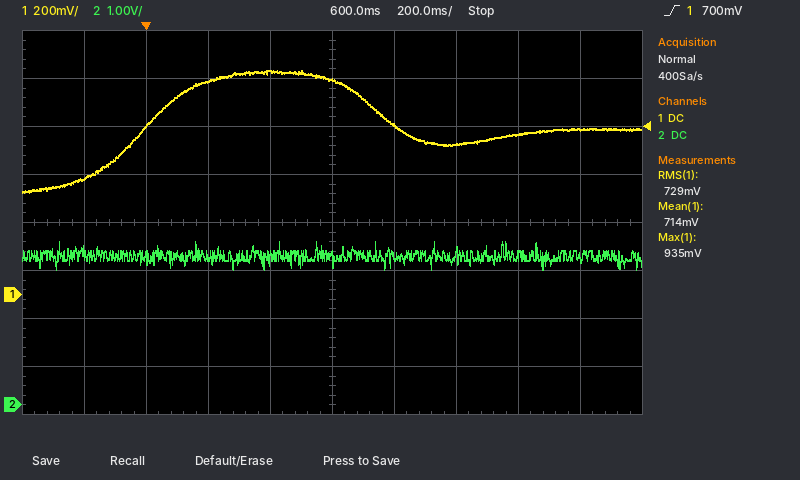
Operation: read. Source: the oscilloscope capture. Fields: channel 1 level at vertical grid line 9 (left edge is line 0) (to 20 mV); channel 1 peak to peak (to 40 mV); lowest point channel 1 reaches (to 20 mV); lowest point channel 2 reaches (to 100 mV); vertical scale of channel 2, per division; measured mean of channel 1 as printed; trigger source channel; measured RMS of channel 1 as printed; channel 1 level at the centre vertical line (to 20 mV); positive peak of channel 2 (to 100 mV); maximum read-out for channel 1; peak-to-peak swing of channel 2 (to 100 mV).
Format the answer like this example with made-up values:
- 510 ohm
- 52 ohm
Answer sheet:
- 680 mV
- 520 mV
- 420 mV
- 2.8 V
- 1 V
- 714 mV
- channel 1
- 729 mV
- 900 mV
- 3.4 V
- 935 mV
- 600 mV
